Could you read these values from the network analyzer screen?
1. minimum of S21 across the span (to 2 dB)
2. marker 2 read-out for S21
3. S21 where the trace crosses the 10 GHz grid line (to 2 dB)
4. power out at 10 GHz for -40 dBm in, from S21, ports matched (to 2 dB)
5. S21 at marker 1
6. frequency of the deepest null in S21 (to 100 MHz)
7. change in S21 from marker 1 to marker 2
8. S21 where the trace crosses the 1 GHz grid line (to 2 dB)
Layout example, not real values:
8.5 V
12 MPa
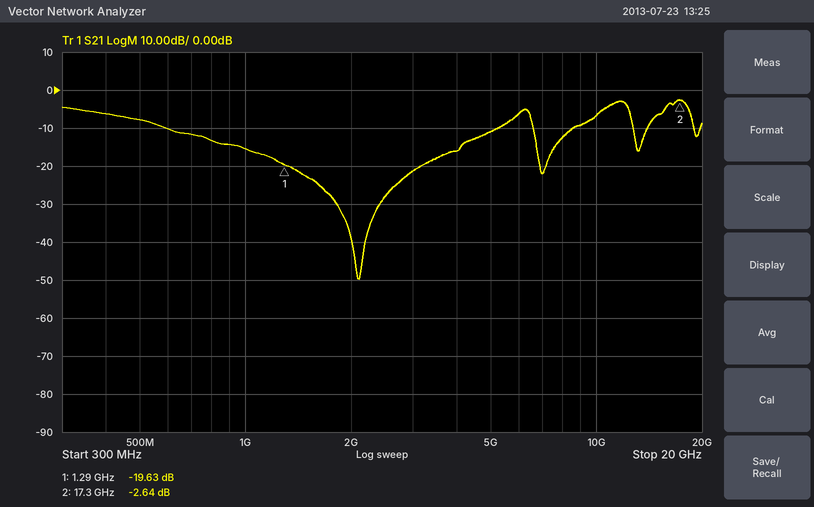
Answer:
-50 dB
-2.64 dB
-6 dB
-46 dBm
-19.63 dB
2.1 GHz
16.99 dB
-16 dB
